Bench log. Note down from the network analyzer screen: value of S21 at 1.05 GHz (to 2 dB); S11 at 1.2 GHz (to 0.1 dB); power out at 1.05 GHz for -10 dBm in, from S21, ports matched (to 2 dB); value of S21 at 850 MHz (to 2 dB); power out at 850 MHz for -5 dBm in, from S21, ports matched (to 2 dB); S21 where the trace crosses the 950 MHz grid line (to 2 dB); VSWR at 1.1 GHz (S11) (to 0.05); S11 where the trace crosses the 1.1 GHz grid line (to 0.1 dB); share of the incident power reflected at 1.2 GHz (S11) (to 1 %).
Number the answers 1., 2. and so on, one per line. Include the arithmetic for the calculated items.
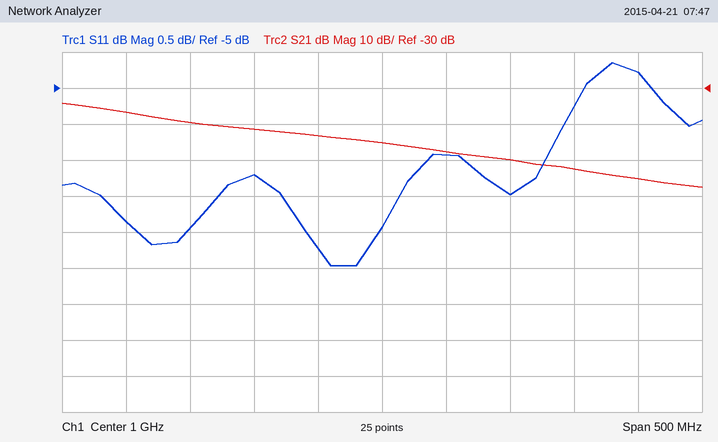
1. -48 dB
2. -4.8 dB
3. -10 dBm + (-48 dB) = -58 dBm
4. -40 dB
5. -5 dBm + (-40 dB) = -44 dBm
6. -44 dB
7. |Γ| = 10^(-6.5/20) = 0.4732; VSWR = (1 + 0.4732)/(1 − 0.4732) ≈ 2.80
8. -6.5 dB
9. 10^(-4.8/10) ≈ 33 %
